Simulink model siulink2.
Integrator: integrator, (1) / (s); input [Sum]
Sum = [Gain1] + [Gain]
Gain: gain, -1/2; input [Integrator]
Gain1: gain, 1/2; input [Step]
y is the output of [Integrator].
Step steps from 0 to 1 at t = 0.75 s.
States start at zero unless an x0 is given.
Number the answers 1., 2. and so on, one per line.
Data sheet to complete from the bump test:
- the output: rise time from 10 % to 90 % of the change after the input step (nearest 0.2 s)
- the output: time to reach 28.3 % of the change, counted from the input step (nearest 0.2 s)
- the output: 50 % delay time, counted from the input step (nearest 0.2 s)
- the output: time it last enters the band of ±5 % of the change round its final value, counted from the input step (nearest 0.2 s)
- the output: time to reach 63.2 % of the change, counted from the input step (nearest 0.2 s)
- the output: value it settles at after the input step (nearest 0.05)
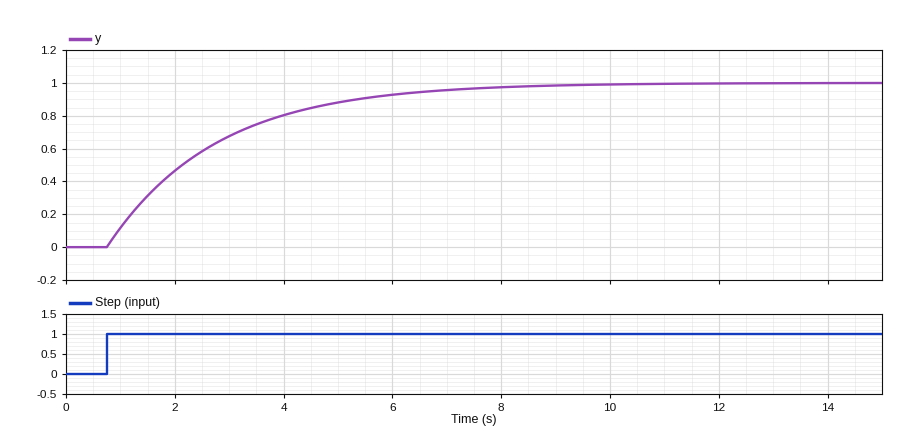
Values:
1. 4.4 s
2. 0.6 s
3. 1.4 s
4. 6.0 s
5. 2.0 s
6. 1.00
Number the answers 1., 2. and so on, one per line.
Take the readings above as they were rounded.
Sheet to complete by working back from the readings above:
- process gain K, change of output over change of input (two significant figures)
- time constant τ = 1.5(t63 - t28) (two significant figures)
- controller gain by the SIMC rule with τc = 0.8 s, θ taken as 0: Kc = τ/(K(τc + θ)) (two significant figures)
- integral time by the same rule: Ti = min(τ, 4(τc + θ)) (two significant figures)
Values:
1. 1.0
2. 2.1 s
3. 2.6
4. 2.1 s
